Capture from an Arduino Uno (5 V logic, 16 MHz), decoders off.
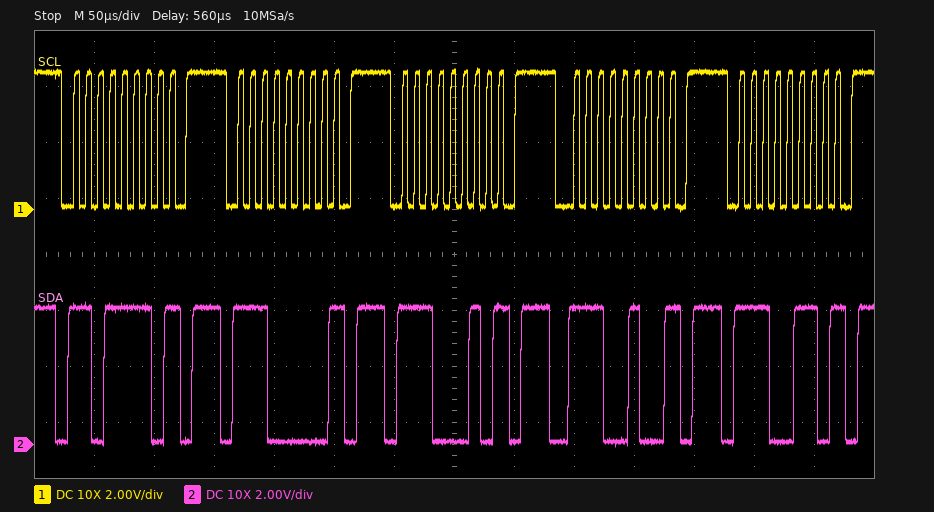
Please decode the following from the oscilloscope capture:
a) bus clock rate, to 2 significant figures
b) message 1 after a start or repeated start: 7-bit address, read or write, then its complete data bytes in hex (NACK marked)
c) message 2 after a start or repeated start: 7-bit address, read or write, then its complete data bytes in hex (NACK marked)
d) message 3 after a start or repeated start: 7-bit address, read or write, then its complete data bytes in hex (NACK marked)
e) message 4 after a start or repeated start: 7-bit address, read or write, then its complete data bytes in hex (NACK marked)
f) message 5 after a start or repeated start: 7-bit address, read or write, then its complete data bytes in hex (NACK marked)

100 kHz
0x6F write NACK
0x70 write NACK
0x71 write NACK
0x72 write NACK
0x73 write NACK
